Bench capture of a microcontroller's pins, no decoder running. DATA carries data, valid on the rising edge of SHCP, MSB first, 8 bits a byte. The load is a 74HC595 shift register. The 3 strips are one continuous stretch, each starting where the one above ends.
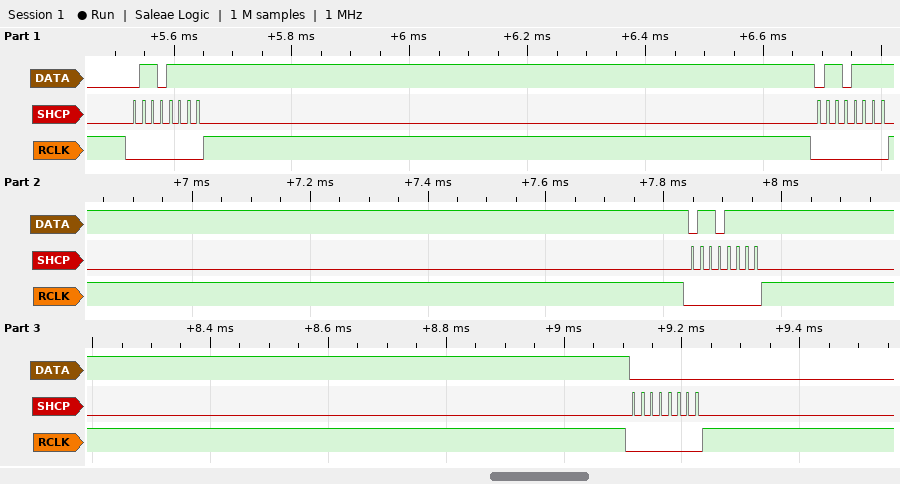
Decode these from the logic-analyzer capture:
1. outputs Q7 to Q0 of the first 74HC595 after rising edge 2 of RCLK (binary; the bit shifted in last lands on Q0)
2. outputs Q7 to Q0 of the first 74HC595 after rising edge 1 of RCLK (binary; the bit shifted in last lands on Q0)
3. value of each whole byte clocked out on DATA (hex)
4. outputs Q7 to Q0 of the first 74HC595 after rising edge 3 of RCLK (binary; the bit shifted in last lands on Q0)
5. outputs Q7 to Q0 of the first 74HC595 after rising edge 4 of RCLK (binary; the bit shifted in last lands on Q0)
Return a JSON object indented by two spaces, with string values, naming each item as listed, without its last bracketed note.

{
  "outputs Q7 to Q0 of the first 74HC595 after rising edge 2 of RCLK": "01101111",
  "outputs Q7 to Q0 of the first 74HC595 after rising edge 1 of RCLK": "01101111",
  "value of each whole byte clocked out on DATA": "0x6F 0x6F 0x6F 0x00",
  "outputs Q7 to Q0 of the first 74HC595 after rising edge 3 of RCLK": "01101111",
  "outputs Q7 to Q0 of the first 74HC595 after rising edge 4 of RCLK": "00000000"
}
